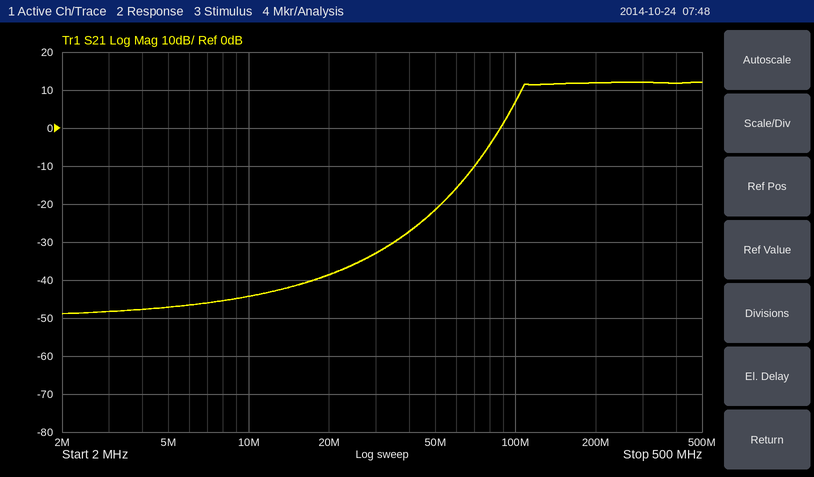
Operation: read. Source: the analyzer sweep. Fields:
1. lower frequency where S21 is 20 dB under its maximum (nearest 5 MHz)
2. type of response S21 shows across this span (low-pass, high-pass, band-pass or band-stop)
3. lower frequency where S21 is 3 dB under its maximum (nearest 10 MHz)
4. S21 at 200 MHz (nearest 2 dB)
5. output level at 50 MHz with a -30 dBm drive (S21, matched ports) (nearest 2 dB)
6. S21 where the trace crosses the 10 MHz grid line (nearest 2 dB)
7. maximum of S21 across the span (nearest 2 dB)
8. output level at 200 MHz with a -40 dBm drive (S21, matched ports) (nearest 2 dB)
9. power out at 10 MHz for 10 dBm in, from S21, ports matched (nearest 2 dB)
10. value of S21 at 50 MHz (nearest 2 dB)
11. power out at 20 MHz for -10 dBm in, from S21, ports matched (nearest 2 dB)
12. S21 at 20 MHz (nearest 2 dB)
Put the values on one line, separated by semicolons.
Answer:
75 MHz; high-pass; 100 MHz; 12 dB; -52 dBm; -44 dB; 12 dB; -28 dBm; -34 dBm; -22 dB; -48 dBm; -38 dB
